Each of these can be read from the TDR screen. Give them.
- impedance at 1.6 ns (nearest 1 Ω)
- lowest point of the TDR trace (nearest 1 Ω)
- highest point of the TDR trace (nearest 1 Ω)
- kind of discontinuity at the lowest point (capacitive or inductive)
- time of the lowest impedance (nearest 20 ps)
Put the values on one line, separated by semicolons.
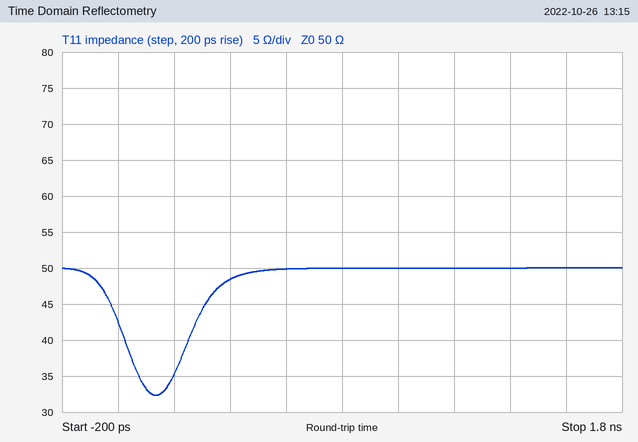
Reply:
50 Ω; 32 Ω; 50 Ω; capacitive; 140 ps
